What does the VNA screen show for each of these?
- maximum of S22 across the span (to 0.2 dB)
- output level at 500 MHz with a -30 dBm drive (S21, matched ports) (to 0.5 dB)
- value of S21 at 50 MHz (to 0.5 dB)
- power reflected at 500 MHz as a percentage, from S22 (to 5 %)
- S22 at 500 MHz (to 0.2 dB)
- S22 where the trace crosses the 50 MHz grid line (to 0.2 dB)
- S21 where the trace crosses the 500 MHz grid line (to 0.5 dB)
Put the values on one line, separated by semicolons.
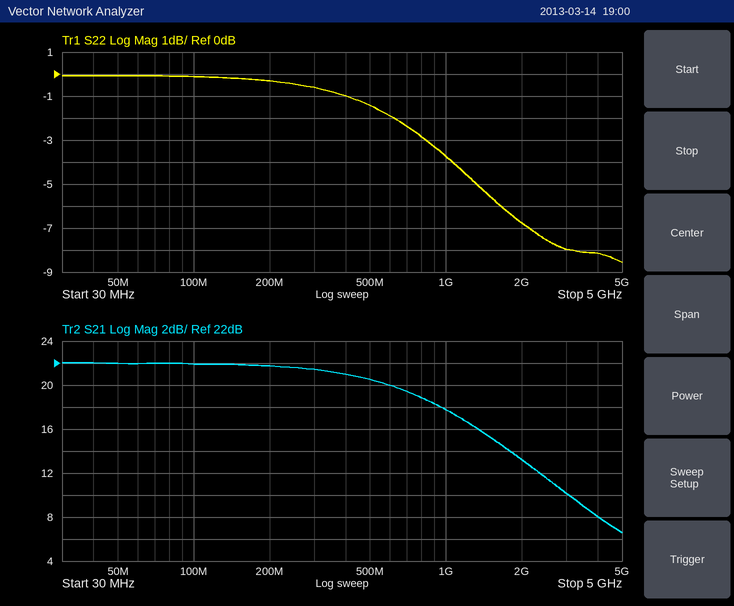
0.0 dB; -9.5 dBm; 22.0 dB; 70 %; -1.4 dB; 0.0 dB; 20.5 dB
